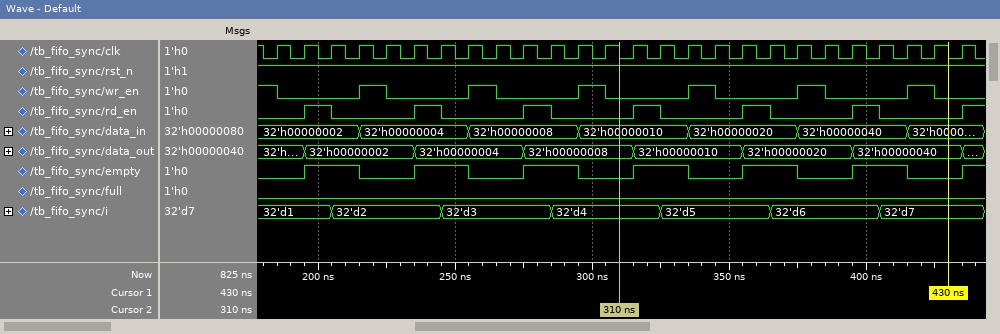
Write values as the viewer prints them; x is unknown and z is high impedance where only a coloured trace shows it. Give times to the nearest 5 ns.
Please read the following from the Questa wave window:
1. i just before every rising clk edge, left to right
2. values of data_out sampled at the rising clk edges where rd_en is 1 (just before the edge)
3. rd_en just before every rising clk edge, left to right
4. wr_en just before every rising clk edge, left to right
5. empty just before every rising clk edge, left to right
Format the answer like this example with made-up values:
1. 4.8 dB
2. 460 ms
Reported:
1. 32'd1, 32'd1, 32'd1, 32'd2, 32'd2, 32'd2, 32'd2, 32'd3, 32'd3, 32'd3, 32'd3, 32'd4, 32'd4, 32'd4, 32'd4, 32'd5, 32'd5, 32'd5, 32'd5, 32'd6, 32'd6, 32'd6, 32'd6, 32'd7, 32'd7, 32'd7
2. 32'h00000002, 32'h00000004, 32'h00000008, 32'h00000010, 32'h00000020, 32'h00000040
3. 0 0 1 0 0 0 1 0 0 0 1 0 0 0 1 0 0 0 1 0 0 0 1 0 0 0
4. 1 0 0 0 1 0 0 0 1 0 0 0 1 0 0 0 1 0 0 0 1 0 0 0 1 0
5. 0 0 1 1 0 0 1 1 0 0 1 1 0 0 1 1 0 0 1 1 0 0 1 1 0 0
